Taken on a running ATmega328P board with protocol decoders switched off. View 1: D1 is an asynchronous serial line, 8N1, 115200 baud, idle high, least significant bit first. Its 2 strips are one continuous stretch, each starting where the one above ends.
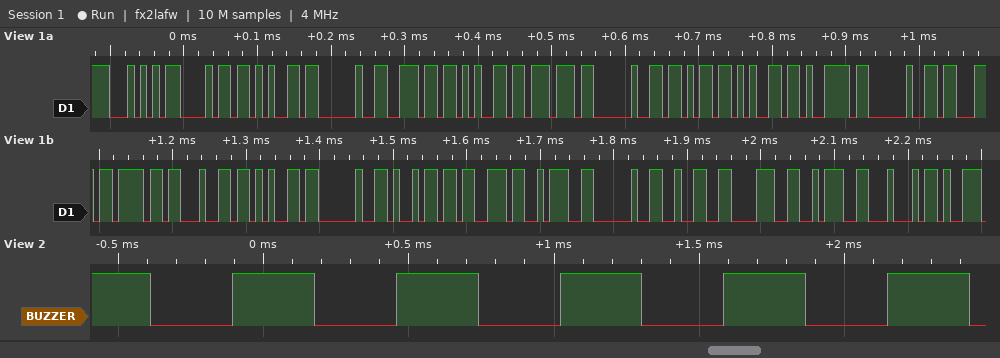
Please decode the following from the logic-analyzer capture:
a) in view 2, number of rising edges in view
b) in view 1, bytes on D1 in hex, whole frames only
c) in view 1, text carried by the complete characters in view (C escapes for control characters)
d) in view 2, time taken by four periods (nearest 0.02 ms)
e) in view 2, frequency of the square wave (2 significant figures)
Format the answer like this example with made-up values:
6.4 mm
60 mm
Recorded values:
5
54 68 65 20 6E 65 77 20 6B 65 79 20 63 6F 64 65 20 69 73 3A 20 32 38 3A 44
"The new key code is: 28:D"
2.24 ms
1.8 kHz
